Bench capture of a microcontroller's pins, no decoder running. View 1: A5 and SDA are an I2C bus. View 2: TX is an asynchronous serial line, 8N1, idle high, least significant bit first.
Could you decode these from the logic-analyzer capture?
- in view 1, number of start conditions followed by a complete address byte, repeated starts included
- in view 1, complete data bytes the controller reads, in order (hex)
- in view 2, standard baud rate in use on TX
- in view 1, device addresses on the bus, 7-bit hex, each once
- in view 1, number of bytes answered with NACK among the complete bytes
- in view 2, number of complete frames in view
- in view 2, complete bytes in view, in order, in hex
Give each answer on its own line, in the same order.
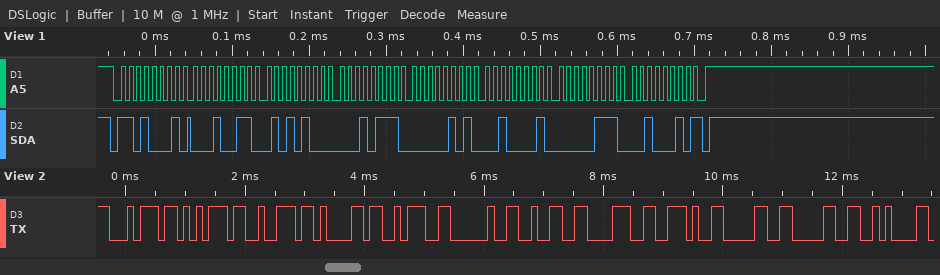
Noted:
1
13 54 17 05 21 07 22
9600 baud
0x68
1
12
0x74 0x75 0x72 0x61 0x3A 0x20 0x32 0x38 0x2E 0x30 0x30 0x0A
